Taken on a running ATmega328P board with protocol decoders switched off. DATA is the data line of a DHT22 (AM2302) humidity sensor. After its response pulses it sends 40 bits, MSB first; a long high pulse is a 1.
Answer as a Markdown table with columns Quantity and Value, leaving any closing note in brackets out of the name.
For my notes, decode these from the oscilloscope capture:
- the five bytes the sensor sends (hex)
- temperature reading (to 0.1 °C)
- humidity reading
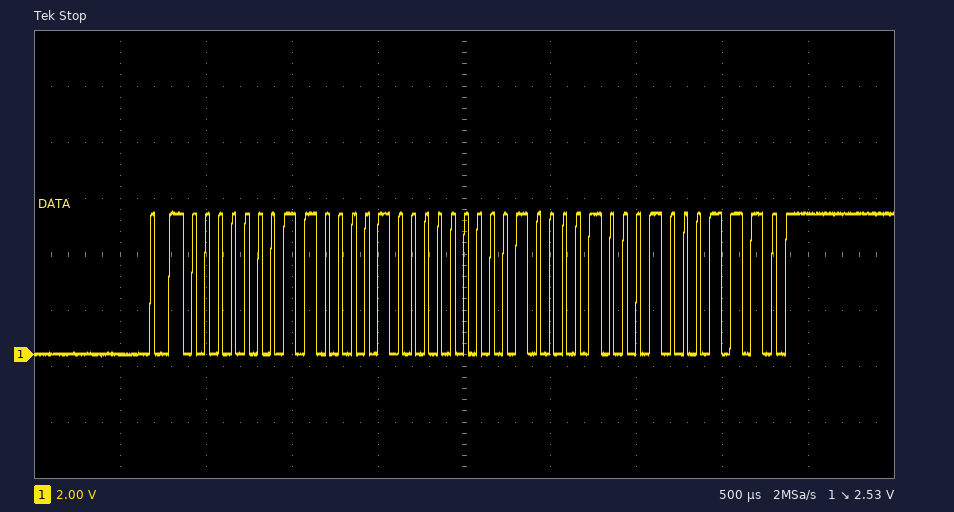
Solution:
| Quantity | Value |
|---|---|
| the five bytes the sensor sends | 01 84 01 08 8E |
| temperature reading | 26.4 °C |
| humidity reading | 38.8 % |
